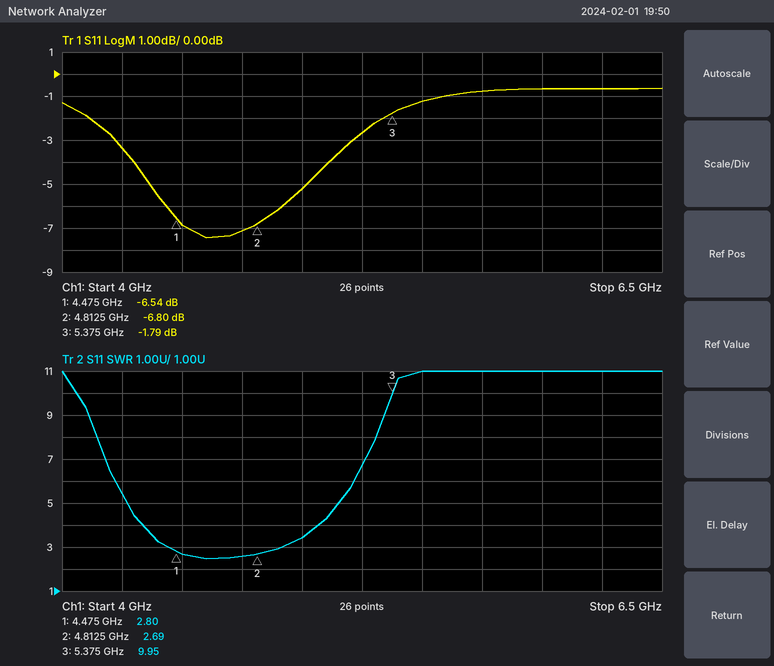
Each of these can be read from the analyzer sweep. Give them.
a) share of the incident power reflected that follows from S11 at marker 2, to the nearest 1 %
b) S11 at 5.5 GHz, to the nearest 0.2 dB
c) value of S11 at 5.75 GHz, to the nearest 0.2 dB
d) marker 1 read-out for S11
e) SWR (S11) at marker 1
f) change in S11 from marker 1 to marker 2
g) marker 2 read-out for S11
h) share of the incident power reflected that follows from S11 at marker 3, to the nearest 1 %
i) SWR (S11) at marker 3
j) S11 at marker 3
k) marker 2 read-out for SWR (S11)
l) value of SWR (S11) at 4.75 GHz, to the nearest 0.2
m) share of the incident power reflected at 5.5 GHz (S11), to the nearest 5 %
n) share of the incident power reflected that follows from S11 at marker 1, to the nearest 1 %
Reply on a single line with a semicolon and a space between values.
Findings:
21 %; -1.2 dB; -0.8 dB; -6.54 dB; 2.80; -0.26 dB; -6.80 dB; 66 %; 9.95; -1.79 dB; 2.69; 2.6; 75 %; 22 %
